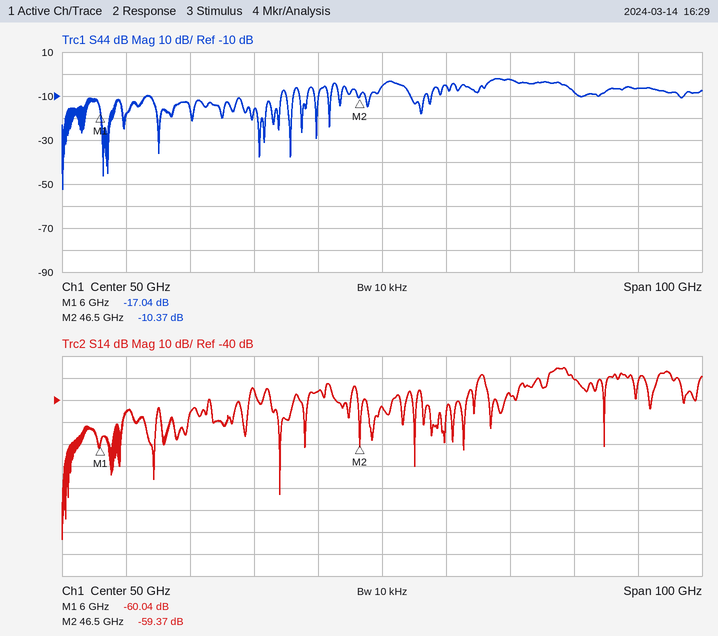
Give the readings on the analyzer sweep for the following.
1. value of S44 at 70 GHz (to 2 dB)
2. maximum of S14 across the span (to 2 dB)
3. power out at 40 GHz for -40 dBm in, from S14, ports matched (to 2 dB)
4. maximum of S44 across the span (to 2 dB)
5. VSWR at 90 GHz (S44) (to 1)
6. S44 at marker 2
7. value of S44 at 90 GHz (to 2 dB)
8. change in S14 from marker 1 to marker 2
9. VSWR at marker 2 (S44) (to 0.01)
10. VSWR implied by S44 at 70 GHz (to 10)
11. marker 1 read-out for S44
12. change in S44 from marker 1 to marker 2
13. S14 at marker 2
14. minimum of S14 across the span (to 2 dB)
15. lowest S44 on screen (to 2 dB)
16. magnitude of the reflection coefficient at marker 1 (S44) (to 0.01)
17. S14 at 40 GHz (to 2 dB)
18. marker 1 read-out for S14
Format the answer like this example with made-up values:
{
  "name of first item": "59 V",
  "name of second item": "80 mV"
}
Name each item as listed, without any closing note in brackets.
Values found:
{
  "value of S44 at 70 GHz": "-2 dB",
  "maximum of S14 across the span": "-26 dB",
  "power out at 40 GHz for -40 dBm in, from S14, ports matched": "-76 dBm",
  "maximum of S44 across the span": "-2 dB",
  "VSWR at 90 GHz (S44)": "3",
  "S44 at marker 2": "-10.37 dB",
  "value of S44 at 90 GHz": "-6 dB",
  "change in S14 from marker 1 to marker 2": "0.67 dB",
  "VSWR at marker 2 (S44)": "1.87",
  "VSWR implied by S44 at 70 GHz": "10",
  "marker 1 read-out for S44": "-17.04 dB",
  "change in S44 from marker 1 to marker 2": "6.67 dB",
  "S14 at marker 2": "-59.37 dB",
  "minimum of S14 across the span": "-104 dB",
  "lowest S44 on screen": "-52 dB",
  "magnitude of the reflection coefficient at marker 1 (S44)": "0.14",
  "S14 at 40 GHz": "-36 dB",
  "marker 1 read-out for S14": "-60.04 dB"
}
